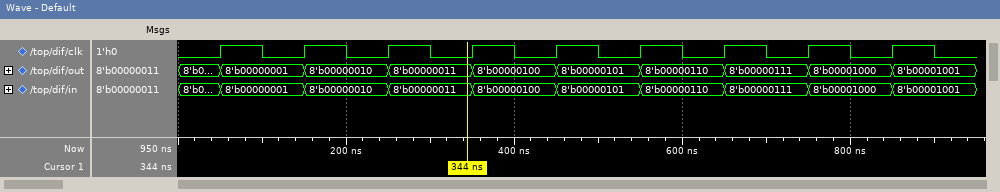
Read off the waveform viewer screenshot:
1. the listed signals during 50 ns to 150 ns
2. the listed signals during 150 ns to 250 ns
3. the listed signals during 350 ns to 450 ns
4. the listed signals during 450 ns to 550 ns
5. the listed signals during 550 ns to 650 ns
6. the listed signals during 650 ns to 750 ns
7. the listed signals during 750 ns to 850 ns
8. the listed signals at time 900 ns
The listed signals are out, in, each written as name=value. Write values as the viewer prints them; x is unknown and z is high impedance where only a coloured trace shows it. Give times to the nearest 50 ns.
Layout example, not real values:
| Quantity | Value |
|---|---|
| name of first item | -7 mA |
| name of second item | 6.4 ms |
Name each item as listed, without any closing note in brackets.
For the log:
| Quantity | Value |
|---|---|
| the listed signals during 50 ns to 150 ns | out=8'b00000001, in=8'b00000001 |
| the listed signals during 150 ns to 250 ns | out=8'b00000010, in=8'b00000010 |
| the listed signals during 350 ns to 450 ns | out=8'b00000100, in=8'b00000100 |
| the listed signals during 450 ns to 550 ns | out=8'b00000101, in=8'b00000101 |
| the listed signals during 550 ns to 650 ns | out=8'b00000110, in=8'b00000110 |
| the listed signals during 650 ns to 750 ns | out=8'b00000111, in=8'b00000111 |
| the listed signals during 750 ns to 850 ns | out=8'b00001000, in=8'b00001000 |
| the listed signals at time 900 ns | out=8'b00001001, in=8'b00001001 |
